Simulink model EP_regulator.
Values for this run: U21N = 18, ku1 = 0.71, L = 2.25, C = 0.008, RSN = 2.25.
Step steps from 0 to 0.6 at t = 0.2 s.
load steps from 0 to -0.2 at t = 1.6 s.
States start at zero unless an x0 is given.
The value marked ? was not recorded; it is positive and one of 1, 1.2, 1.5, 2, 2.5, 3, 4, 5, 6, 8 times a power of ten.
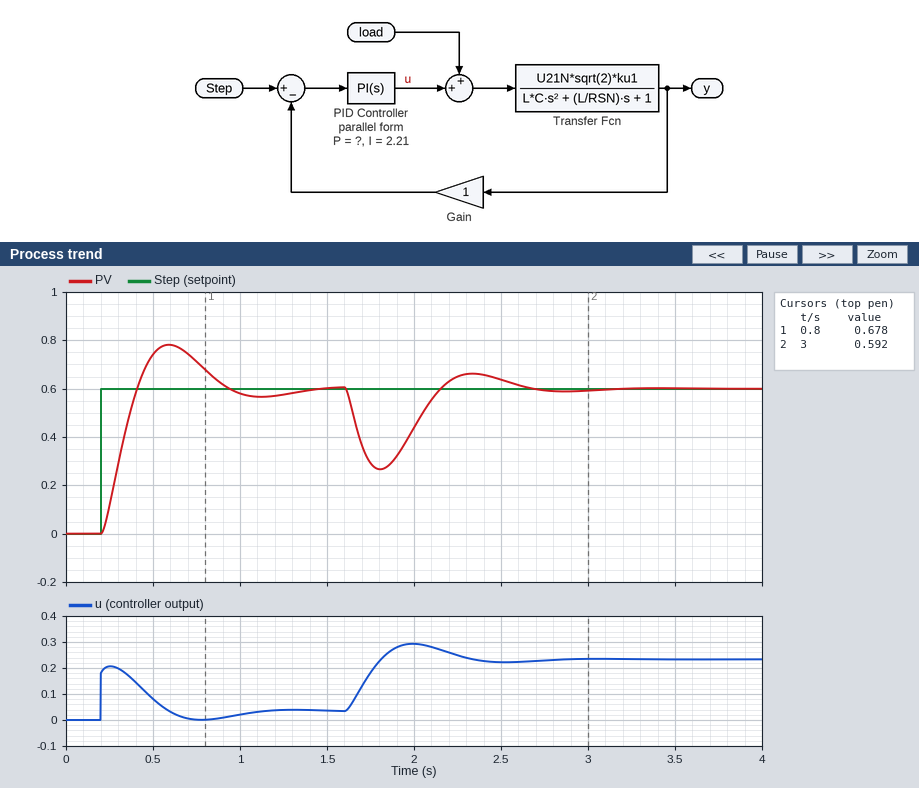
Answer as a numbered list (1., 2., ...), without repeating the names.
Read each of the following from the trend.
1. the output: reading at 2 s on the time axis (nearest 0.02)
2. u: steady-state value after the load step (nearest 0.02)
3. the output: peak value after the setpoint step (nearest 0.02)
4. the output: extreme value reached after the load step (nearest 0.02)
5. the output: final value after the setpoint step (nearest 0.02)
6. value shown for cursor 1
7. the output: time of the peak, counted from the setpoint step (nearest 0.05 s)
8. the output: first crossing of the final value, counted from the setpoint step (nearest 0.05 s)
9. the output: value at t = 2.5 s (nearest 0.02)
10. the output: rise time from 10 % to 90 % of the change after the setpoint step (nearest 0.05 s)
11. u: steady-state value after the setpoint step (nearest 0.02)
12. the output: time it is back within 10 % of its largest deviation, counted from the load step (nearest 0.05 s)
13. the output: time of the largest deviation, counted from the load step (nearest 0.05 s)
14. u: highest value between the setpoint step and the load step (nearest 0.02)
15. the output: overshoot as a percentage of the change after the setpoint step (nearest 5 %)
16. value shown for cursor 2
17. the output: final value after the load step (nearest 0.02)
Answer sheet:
1. 0.44
2. 0.24
3. 0.78
4. 0.26
5. 0.60
6. 0.678
7. 0.40 s
8. 0.20 s
9. 0.64
10. 0.15 s
11. 0.04
12. 0.90 s
13. 0.20 s
14. 0.20
15. 30 %
16. 0.592
17. 0.60
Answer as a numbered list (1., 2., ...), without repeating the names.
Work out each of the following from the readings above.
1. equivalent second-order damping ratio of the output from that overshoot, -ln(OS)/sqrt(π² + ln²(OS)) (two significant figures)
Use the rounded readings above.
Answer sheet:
1. 0.36
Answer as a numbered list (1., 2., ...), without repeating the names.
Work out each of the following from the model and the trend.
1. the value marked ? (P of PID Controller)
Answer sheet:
1. 0.3
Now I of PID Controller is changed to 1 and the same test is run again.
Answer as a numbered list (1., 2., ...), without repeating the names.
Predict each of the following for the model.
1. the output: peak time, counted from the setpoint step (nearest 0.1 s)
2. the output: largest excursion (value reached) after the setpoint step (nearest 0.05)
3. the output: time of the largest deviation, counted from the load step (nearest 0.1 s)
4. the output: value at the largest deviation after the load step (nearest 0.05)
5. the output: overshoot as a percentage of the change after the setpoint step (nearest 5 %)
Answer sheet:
1. 0.5 s
2. 0.70
3. 0.3 s
4. 0.20
5. 15 %
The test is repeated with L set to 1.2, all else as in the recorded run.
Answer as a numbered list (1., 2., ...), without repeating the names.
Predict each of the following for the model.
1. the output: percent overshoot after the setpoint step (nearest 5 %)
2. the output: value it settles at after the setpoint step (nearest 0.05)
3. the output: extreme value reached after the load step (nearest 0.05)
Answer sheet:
1. 20 %
2. 0.60
3. 0.20
